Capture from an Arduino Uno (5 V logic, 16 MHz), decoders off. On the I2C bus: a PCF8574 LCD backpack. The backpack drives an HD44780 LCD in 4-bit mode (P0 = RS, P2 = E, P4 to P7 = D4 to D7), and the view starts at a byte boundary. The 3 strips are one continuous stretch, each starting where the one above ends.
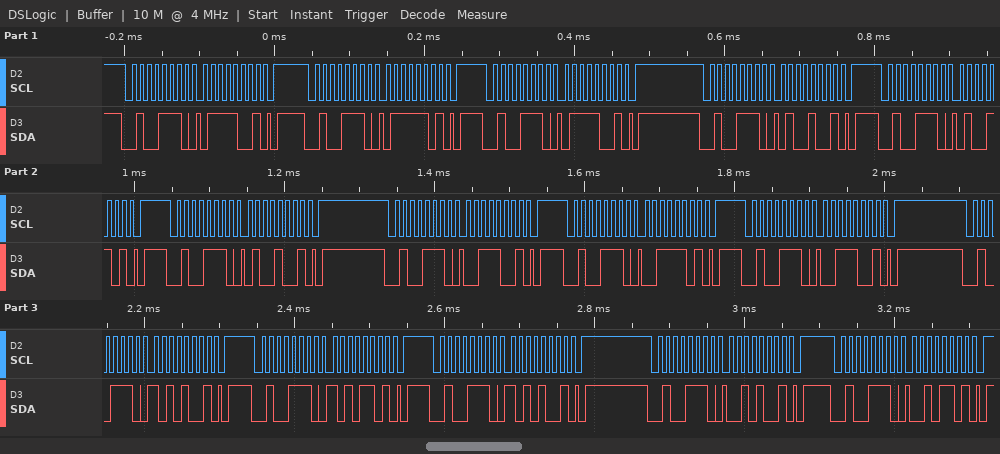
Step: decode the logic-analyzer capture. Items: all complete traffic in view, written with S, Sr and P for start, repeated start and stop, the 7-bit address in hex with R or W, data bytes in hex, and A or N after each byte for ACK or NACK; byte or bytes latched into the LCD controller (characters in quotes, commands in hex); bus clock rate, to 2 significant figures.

S 27W A 79 A P S 27W A 7D A P S 27W A 79 A P S 27W A 49 A P S 27W A 4D A P S 27W A 49 A P S 27W A 39 A P S 27W A 3D A P S 27W A 39 A P S 27W A A9 A P S 27W A AD A P S 27W A A9 A P S 27W A 29 A P S 27W A 2D A P
't' ':'
100 kHz
